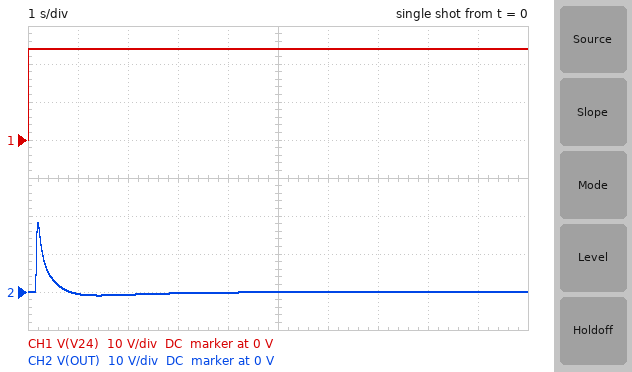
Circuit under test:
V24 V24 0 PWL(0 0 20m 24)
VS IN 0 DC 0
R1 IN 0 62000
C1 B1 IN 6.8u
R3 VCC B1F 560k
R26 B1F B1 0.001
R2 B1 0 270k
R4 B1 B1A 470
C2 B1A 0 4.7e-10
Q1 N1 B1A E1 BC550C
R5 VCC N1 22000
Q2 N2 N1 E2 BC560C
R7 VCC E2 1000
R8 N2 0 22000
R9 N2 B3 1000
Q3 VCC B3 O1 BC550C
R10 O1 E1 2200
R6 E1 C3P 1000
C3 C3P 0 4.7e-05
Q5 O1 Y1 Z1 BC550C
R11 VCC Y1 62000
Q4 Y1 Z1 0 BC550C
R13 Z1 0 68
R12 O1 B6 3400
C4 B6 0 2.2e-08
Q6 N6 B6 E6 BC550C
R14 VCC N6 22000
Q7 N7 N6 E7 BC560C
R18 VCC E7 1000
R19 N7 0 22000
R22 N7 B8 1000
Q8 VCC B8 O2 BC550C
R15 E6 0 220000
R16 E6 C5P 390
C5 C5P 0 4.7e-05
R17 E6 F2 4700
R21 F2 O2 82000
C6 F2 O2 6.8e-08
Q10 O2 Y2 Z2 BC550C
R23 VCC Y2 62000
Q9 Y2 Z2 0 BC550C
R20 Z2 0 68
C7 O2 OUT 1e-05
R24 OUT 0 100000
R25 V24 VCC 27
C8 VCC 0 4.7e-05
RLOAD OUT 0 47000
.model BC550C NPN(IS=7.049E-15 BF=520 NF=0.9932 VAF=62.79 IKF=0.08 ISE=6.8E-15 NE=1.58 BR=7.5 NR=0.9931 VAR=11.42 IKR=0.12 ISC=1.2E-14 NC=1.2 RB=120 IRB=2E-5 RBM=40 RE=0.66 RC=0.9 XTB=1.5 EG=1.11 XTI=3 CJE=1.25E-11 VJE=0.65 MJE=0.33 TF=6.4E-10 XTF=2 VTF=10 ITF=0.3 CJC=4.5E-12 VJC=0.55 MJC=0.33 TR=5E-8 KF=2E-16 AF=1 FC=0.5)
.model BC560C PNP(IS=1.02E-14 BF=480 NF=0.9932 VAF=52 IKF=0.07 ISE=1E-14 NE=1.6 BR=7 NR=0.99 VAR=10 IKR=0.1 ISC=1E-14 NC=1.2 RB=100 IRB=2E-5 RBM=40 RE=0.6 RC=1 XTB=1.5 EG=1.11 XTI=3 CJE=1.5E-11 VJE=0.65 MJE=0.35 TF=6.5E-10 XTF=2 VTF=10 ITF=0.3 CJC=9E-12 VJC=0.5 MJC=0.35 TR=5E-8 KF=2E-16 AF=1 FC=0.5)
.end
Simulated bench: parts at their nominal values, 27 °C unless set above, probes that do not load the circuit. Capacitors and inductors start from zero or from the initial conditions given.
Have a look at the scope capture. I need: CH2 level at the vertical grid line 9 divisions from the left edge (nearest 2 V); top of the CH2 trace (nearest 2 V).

0 V
18 V
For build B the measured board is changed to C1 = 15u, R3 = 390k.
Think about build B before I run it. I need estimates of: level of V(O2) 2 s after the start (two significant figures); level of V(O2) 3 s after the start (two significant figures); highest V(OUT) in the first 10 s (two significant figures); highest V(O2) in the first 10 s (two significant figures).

8.6 V
8.2 V
9.4 V
11 V
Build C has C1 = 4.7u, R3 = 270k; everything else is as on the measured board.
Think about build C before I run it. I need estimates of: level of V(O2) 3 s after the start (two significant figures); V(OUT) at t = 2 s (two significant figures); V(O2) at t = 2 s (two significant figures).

10 V
-1.5 V
12 V
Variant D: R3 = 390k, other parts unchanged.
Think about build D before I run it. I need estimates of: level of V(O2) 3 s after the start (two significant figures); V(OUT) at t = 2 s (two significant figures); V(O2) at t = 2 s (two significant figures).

8.6 V
-1.1 V
10 V
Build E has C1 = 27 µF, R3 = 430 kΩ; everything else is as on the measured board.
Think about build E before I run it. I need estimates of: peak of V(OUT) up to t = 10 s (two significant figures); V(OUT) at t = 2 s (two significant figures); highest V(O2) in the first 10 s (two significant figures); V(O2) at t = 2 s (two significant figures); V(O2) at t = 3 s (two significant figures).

3.0 V
210 mV
6.5 V
4.7 V
5.1 V
